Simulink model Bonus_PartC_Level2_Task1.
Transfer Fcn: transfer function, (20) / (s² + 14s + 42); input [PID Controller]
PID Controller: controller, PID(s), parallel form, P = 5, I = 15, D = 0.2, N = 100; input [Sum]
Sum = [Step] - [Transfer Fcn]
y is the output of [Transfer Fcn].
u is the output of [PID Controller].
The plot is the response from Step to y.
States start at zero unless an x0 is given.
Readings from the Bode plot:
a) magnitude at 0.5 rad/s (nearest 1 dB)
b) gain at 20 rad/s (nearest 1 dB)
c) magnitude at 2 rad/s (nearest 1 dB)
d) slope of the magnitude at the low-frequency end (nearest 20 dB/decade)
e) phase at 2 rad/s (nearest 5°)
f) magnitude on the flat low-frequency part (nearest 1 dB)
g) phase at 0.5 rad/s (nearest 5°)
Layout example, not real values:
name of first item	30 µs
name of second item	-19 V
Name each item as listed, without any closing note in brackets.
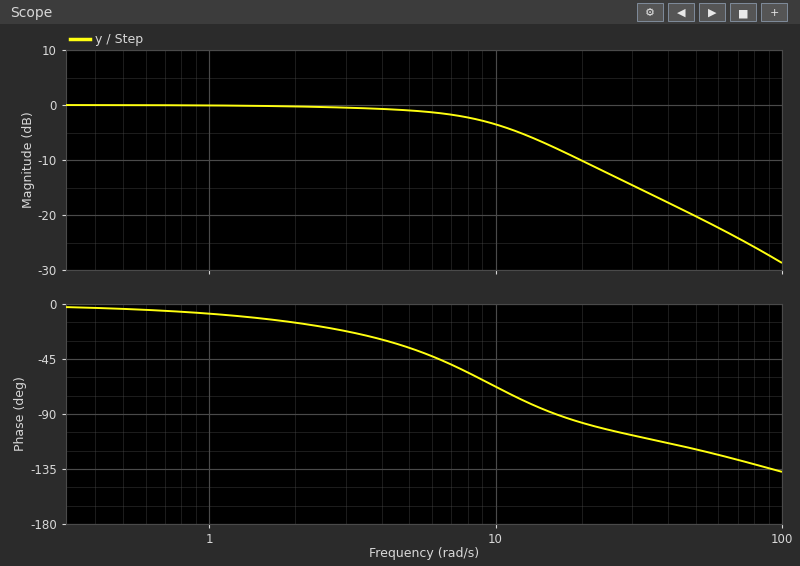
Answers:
magnitude at 0.5 rad/s	0 dB
gain at 20 rad/s	-10 dB
magnitude at 2 rad/s	0 dB
slope of the magnitude at the low-frequency end	0 dB/decade
phase at 2 rad/s	-15°
magnitude on the flat low-frequency part	0 dB
phase at 0.5 rad/s	-5°
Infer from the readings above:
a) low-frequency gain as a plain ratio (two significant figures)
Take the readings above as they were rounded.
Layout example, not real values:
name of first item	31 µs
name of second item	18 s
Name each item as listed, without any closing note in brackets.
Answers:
low-frequency gain as a plain ratio	1.0
